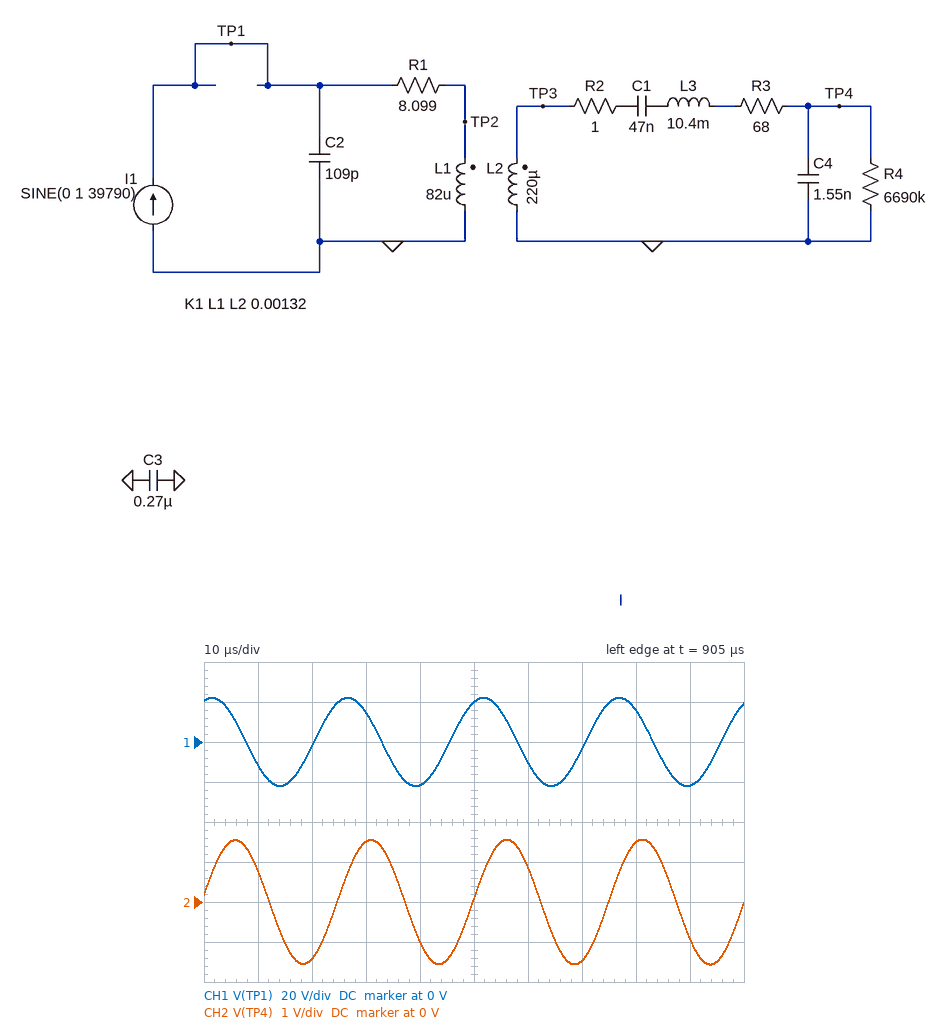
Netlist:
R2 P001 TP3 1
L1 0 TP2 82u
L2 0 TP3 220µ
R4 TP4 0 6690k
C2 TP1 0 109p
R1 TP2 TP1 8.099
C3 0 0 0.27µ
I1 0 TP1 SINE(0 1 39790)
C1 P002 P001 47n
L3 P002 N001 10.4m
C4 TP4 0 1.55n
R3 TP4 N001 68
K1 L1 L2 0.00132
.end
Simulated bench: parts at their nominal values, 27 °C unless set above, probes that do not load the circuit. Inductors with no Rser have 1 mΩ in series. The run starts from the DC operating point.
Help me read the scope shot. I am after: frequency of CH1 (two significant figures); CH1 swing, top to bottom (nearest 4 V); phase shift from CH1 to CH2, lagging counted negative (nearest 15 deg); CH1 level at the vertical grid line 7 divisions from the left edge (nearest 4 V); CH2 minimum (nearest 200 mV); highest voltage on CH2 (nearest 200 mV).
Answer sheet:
40 kHz
44 V
-60 deg
-4 V
-1.6 V
1.6 V
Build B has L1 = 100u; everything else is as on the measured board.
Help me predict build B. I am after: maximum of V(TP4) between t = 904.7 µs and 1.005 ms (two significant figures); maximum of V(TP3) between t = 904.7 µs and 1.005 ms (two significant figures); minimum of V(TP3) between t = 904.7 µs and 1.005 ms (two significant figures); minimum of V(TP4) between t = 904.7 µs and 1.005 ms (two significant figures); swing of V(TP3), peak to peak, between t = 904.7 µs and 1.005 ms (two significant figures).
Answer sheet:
1.7 V
65 mV
-65 mV
-1.7 V
130 mV
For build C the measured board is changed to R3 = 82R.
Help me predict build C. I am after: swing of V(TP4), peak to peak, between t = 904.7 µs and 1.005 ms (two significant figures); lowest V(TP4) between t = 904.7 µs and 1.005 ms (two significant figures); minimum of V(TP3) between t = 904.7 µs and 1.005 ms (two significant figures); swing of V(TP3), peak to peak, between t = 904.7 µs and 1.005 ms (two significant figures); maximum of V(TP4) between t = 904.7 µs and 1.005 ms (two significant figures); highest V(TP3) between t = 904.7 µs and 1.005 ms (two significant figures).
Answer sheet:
2.7 V
-1.3 V
-55 mV
110 mV
1.3 V
55 mV
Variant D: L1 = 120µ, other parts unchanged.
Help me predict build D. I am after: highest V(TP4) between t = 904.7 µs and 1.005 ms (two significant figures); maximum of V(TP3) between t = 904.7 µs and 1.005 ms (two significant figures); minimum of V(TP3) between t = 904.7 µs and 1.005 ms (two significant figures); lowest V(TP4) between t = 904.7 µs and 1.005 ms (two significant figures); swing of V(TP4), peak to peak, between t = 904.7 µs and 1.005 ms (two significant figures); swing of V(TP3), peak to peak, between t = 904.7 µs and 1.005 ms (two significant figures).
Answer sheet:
1.9 V
71 mV
-71 mV
-1.9 V
3.8 V
140 mV
